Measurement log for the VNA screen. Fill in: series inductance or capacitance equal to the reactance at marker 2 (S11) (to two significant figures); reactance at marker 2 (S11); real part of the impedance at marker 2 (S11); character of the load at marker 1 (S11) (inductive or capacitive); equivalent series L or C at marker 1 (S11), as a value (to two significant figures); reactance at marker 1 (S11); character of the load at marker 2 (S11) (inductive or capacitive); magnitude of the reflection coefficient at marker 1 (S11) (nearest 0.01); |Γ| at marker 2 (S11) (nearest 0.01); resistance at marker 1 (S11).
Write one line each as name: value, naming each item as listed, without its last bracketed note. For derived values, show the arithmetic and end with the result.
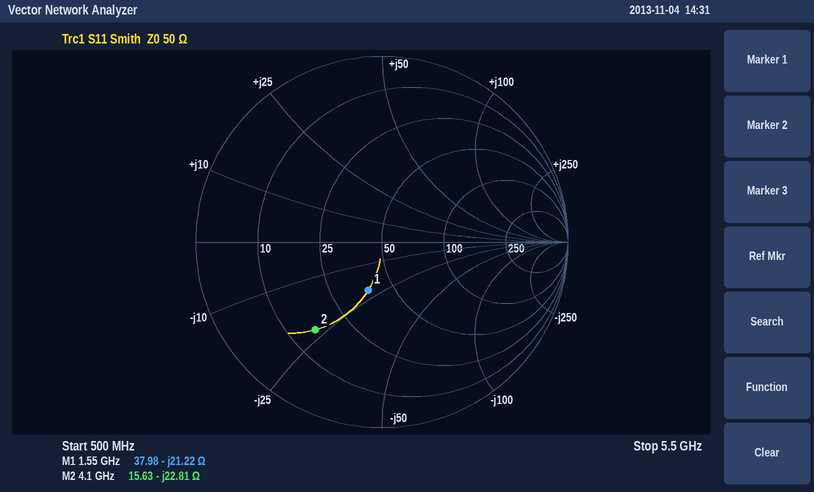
series inductance or capacitance equal to the reactance at marker 2 (S11): C = 1/(2π × 4.1 GHz × 22.81 Ω) ≈ 1.7 pF
reactance at marker 2: -22.81 Ω
real part of the impedance at marker 2: 15.63 Ω
character of the load at marker 1 (S11): capacitive
equivalent series L or C at marker 1 (S11), as a value: C = 1/(2π × 1.55 GHz × 21.22 Ω) ≈ 4.8 pF
reactance at marker 1: -21.22 Ω
character of the load at marker 2 (S11): capacitive
magnitude of the reflection coefficient at marker 1 (S11): 0.27
|Γ| at marker 2 (S11): 0.59
resistance at marker 1: 37.98 Ω
